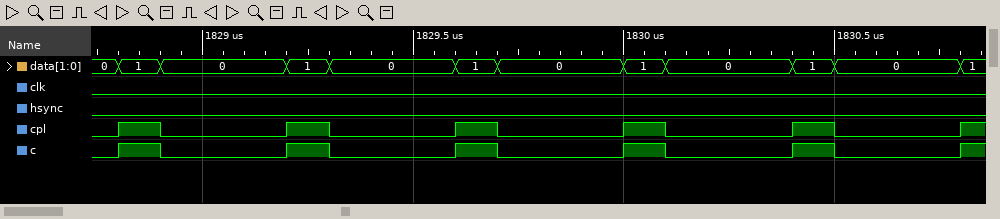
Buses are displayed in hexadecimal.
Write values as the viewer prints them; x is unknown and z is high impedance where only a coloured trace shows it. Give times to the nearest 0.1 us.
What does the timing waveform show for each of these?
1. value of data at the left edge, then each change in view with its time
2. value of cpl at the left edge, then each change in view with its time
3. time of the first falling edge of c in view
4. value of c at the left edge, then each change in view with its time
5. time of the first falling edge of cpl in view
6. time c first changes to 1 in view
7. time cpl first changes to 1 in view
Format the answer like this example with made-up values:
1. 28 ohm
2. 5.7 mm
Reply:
1. 0, 1 at 1828.8 us, 0 at 1828.9 us, 1 at 1829.2 us, 0 at 1829.3 us, 1 at 1829.6 us, 0 at 1829.7 us, 1 at 1830 us, 0 at 1830.1 us, 1 at 1830.4 us, 0 at 1830.5 us, 1 at 1830.8 us
2. 0, 1 at 1828.8 us, 0 at 1828.9 us, 1 at 1829.2 us, 0 at 1829.3 us, 1 at 1829.6 us, 0 at 1829.7 us, 1 at 1830 us, 0 at 1830.1 us, 1 at 1830.4 us, 0 at 1830.5 us, 1 at 1830.8 us
3. 1828.9 us
4. 0, 1 at 1828.8 us, 0 at 1828.9 us, 1 at 1829.2 us, 0 at 1829.3 us, 1 at 1829.6 us, 0 at 1829.7 us, 1 at 1830 us, 0 at 1830.1 us, 1 at 1830.4 us, 0 at 1830.5 us, 1 at 1830.8 us
5. 1828.9 us
6. 1828.8 us
7. 1828.8 us
